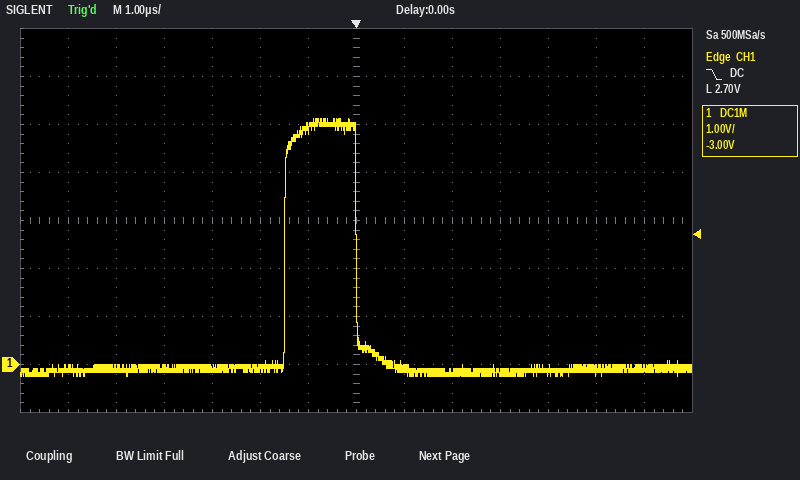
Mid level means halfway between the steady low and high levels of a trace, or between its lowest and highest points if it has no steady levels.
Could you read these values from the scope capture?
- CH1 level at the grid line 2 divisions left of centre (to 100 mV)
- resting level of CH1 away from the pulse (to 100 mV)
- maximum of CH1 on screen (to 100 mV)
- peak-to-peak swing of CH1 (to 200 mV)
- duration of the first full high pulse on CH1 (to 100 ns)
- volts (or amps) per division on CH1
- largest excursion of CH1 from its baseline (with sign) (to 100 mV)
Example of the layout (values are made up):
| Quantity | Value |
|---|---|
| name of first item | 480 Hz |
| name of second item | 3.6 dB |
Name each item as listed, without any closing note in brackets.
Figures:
| Quantity | Value |
|---|---|
| CH1 level at the grid line 2 divisions left of centre | -100 mV |
| resting level of CH1 away from the pulse | -100 mV |
| maximum of CH1 on screen | 5.1 V |
| peak-to-peak swing of CH1 | 5.4 V |
| duration of the first full high pulse on CH1 | 1.5 µs |
| volts (or amps) per division on CH1 | 1 V |
| largest excursion of CH1 from its baseline (with sign) | +5.2 V |
